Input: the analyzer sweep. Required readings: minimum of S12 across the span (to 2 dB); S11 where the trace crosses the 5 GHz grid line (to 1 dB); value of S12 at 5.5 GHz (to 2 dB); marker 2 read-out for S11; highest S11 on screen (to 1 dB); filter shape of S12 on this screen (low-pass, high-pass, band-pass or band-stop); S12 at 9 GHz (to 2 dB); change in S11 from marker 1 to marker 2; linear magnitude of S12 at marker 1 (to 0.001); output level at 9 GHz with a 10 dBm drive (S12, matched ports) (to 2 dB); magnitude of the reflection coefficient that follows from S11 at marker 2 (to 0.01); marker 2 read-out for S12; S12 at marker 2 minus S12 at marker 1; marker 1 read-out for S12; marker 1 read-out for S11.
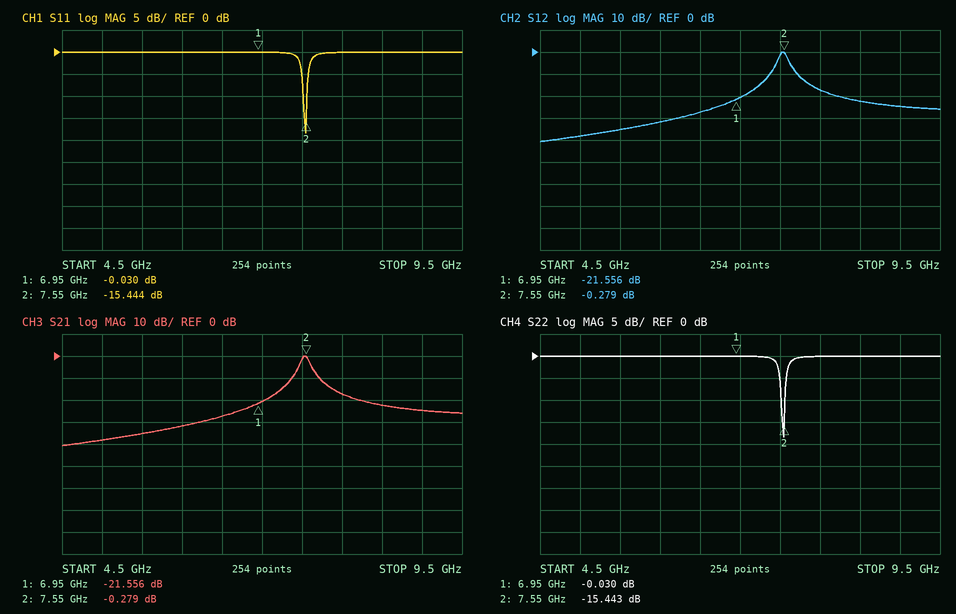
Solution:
-40 dB
0 dB
-36 dB
-15.444 dB
0 dB
band-pass
-24 dB
-15.414 dB
0.084
-14 dBm
0.17
-0.279 dB
21.277 dB
-21.556 dB
-0.030 dB
